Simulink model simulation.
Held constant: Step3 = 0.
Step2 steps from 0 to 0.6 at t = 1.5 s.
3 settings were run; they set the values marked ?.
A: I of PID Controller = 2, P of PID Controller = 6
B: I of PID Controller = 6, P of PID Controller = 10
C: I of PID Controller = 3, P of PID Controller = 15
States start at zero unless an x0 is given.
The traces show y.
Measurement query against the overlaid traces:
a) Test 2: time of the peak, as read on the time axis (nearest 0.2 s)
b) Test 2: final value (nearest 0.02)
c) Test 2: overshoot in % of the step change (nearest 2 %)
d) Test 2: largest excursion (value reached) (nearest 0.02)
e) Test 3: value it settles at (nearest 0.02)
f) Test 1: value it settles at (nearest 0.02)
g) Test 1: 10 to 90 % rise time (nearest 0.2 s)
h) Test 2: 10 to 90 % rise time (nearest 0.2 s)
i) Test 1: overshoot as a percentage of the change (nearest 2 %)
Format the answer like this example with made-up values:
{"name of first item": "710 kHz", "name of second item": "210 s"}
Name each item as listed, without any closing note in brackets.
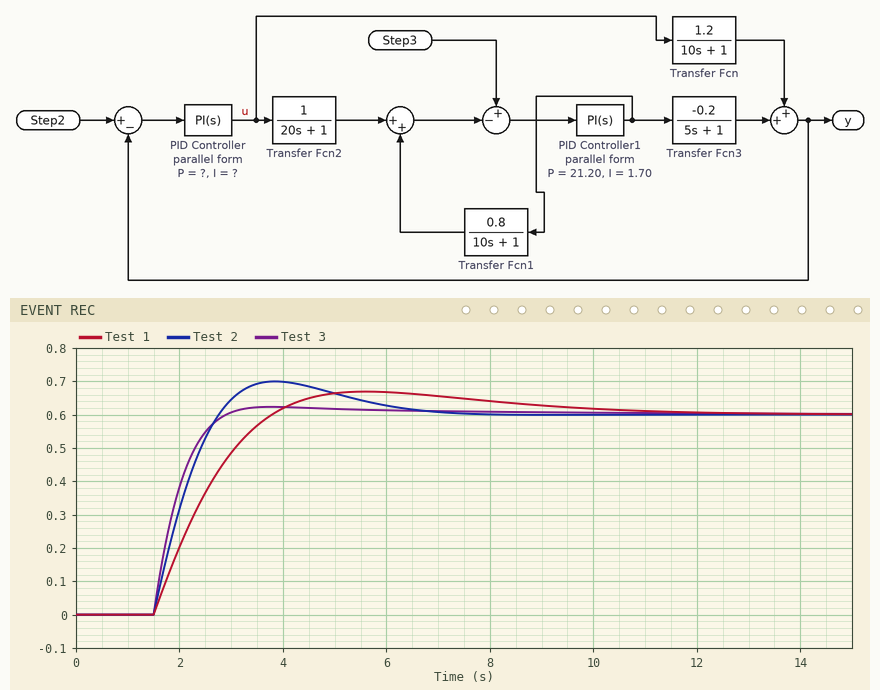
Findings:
{"Test 2: time of the peak, as read on the time axis": "3.8 s", "Test 2: final value": "0.60", "Test 2: overshoot in % of the step change": "16 %", "Test 2: largest excursion (value reached)": "0.70", "Test 3: value it settles at": "0.60", "Test 1: value it settles at": "0.60", "Test 1: 10 to 90 % rise time": "1.6 s", "Test 2: 10 to 90 % rise time": "1.0 s", "Test 1: overshoot as a percentage of the change": "12 %"}
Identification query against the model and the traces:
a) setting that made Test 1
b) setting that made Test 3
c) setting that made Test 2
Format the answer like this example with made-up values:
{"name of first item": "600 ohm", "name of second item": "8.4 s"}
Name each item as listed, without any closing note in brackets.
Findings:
{"setting that made Test 1": "A", "setting that made Test 3": "C", "setting that made Test 2": "B"}
